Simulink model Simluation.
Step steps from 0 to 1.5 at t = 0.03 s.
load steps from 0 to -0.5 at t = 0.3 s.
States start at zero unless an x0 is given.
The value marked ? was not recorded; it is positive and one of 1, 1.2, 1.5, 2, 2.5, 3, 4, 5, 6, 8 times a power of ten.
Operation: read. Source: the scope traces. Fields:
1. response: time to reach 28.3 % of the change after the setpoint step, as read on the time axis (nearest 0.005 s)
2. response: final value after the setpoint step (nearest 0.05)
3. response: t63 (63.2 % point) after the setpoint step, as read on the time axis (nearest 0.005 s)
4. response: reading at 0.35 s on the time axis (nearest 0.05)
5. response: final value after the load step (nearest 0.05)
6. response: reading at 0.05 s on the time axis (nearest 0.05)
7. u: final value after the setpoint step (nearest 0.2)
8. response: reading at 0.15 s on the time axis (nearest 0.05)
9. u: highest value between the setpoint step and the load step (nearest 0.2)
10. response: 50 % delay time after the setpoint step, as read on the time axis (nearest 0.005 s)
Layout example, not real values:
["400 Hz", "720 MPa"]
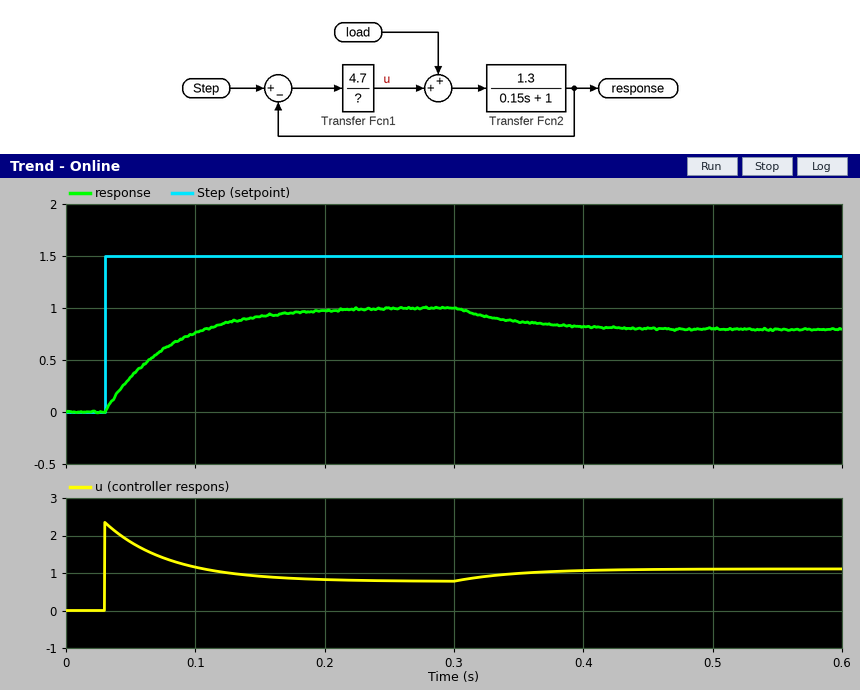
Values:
["0.045 s", "1.00", "0.080 s", "0.85", "0.80", "0.35", "0.8", "0.90", "2.4", "0.065 s"]
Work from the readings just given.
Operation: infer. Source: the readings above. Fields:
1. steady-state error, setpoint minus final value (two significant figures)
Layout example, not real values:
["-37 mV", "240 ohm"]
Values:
["0.50"]
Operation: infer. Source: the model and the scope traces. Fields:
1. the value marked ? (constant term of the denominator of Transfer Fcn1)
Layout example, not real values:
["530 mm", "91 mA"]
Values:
["3"]
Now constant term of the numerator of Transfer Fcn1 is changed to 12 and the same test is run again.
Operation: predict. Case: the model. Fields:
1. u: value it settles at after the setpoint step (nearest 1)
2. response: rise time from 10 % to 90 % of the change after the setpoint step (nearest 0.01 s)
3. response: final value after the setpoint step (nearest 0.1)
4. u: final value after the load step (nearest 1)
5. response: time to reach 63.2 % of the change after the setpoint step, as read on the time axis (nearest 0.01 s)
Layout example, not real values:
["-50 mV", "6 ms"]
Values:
["1", "0.05 s", "1.3", "1", "0.05 s"]
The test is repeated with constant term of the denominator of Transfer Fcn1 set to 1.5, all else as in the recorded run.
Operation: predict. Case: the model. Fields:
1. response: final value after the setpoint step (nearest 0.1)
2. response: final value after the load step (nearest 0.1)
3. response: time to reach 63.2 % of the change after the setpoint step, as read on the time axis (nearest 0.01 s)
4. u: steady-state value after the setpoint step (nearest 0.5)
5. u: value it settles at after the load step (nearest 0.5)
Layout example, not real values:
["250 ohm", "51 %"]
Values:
["1.2", "1.1", "0.06 s", "1.0", "1.5"]
